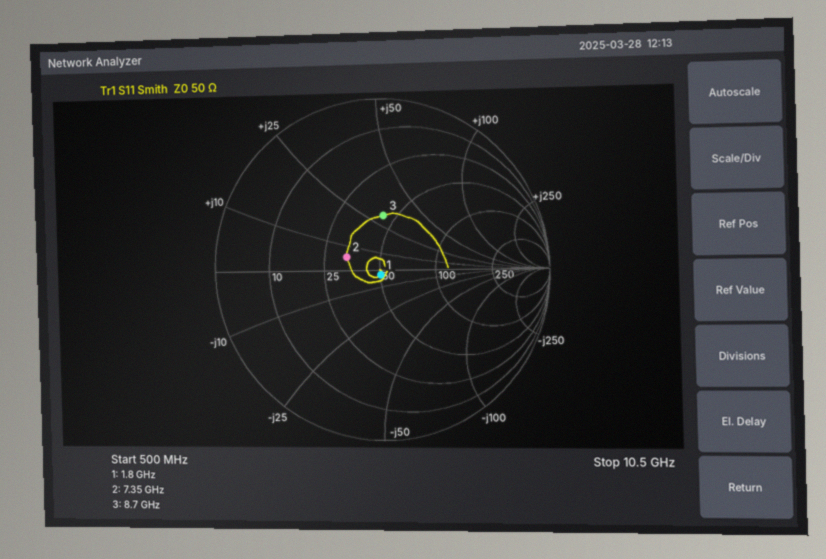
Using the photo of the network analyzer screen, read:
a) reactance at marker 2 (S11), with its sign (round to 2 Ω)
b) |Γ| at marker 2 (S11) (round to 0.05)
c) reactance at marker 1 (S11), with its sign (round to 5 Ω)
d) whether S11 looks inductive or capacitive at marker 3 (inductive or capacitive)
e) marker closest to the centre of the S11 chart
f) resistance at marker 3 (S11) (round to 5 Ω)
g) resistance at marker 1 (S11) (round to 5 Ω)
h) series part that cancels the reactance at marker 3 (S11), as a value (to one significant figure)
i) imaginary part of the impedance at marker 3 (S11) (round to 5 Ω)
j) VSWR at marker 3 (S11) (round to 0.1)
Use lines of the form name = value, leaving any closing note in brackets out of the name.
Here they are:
reactance at marker 2 (S11), with its sign = +6 Ω
|Γ| at marker 2 (S11) = 0.20
reactance at marker 1 (S11), with its sign = -5 Ω
whether S11 looks inductive or capacitive at marker 3 = inductive
marker closest to the centre of the S11 chart = marker 1
resistance at marker 3 (S11) = 45 Ω
resistance at marker 1 (S11) = 50 Ω
series part that cancels the reactance at marker 3 (S11), as a value = 600 fF
imaginary part of the impedance at marker 3 (S11) = +30 Ω
VSWR at marker 3 (S11) = 1.9
